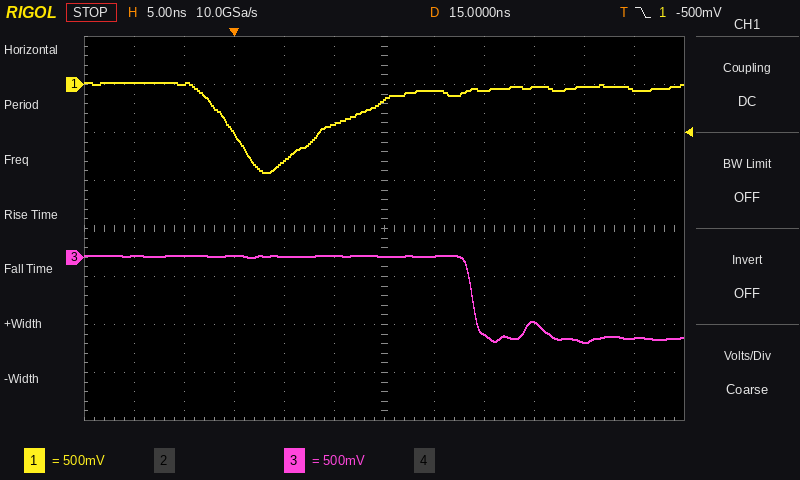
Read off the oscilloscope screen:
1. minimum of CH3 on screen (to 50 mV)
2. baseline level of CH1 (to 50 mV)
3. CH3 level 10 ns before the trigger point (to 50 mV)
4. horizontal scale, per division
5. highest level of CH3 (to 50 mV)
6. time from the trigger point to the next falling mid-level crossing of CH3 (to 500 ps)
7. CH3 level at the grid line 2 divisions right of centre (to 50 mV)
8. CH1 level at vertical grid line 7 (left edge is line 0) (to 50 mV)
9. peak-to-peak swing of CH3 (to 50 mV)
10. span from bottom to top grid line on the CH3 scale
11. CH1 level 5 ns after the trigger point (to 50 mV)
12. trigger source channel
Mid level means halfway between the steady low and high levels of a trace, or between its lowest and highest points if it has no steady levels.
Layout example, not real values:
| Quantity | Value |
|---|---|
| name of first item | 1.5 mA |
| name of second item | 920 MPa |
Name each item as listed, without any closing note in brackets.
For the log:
| Quantity | Value |
|---|---|
| minimum of CH3 on screen | -900 mV |
| baseline level of CH1 | -50 mV |
| CH3 level 10 ns before the trigger point | 0 mV |
| horizontal scale, per division | 5 ns |
| highest level of CH3 | 0 mV |
| time from the trigger point to the next falling mid-level crossing of CH3 | 24.0 ns |
| CH3 level at the grid line 2 divisions right of centre | -800 mV |
| CH1 level at vertical grid line 7 (left edge is line 0) | -50 mV |
| peak-to-peak swing of CH3 | 900 mV |
| span from bottom to top grid line on the CH3 scale | 4 V |
| CH1 level 5 ns after the trigger point | -800 mV |
| trigger source channel | CH1 |
